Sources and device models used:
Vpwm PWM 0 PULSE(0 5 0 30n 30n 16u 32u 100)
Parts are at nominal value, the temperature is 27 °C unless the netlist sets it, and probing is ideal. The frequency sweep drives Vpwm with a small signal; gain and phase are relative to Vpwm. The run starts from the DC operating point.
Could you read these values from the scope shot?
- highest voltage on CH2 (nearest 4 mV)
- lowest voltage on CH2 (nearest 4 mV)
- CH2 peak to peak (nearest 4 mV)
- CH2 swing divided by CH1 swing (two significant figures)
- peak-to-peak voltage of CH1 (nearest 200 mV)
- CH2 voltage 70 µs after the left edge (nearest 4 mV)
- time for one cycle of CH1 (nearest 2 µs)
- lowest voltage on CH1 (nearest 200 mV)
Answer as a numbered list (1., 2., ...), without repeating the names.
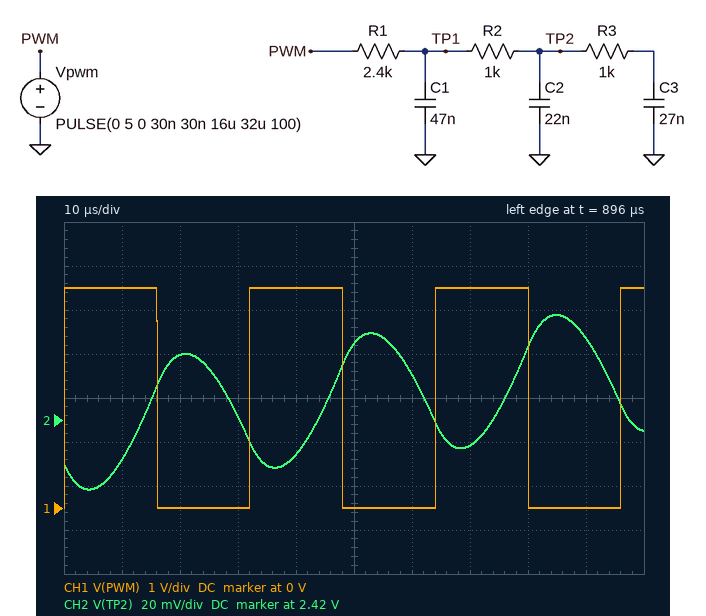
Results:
1. 2.468 V
2. 2.388 V
3. 80 mV
4. 0.016
5. 5.0 V
6. 2.408 V
7. 32 µs
8. 0 V
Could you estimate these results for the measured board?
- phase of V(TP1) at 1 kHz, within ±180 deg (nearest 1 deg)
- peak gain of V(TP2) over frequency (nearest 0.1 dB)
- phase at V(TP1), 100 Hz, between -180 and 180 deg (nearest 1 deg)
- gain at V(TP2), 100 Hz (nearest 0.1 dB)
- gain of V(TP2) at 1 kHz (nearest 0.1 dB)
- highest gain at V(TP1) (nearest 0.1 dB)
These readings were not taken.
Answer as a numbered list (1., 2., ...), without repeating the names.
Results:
1. -47 deg
2. 0 dB
3. -8 deg
4. -0.1 dB
5. -5.9 dB
6. 0 dB
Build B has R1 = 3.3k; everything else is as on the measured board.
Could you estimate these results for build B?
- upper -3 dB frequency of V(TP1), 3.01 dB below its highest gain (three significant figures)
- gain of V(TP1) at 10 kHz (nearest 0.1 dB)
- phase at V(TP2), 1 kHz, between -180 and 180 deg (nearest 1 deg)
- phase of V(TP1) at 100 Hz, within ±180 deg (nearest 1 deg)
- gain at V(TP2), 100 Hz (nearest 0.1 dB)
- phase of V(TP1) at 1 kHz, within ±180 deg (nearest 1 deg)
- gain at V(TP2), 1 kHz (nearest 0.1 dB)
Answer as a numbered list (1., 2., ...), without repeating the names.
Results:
1. 464 Hz
2. -21.0 dB
3. -70 deg
4. -11 deg
5. -0.2 dB
6. -54 deg
7. -7.8 dB
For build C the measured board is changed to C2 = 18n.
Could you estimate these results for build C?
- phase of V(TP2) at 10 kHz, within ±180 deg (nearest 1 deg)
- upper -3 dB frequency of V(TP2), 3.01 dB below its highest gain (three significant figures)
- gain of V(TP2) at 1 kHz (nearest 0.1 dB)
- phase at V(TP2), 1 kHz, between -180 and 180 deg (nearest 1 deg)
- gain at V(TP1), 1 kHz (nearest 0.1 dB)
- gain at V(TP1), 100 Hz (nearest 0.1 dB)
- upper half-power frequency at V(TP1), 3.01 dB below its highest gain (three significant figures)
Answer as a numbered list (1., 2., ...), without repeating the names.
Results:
1. -113 deg
2. 621 Hz
3. -5.6 dB
4. -62 deg
5. -5.0 dB
6. -0.1 dB
7. 656 Hz
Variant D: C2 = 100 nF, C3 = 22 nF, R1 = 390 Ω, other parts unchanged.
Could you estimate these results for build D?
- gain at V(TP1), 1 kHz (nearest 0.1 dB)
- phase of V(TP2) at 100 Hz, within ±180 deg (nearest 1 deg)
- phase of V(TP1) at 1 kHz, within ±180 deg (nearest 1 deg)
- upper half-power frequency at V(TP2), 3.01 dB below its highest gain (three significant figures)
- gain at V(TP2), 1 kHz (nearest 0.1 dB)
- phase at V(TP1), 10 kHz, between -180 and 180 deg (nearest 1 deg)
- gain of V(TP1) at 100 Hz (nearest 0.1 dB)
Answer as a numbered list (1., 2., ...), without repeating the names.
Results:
1. -1.5 dB
2. -7 deg
3. -15 deg
4. 887 Hz
5. -3.6 dB
6. -41 deg
7. 0 dB
